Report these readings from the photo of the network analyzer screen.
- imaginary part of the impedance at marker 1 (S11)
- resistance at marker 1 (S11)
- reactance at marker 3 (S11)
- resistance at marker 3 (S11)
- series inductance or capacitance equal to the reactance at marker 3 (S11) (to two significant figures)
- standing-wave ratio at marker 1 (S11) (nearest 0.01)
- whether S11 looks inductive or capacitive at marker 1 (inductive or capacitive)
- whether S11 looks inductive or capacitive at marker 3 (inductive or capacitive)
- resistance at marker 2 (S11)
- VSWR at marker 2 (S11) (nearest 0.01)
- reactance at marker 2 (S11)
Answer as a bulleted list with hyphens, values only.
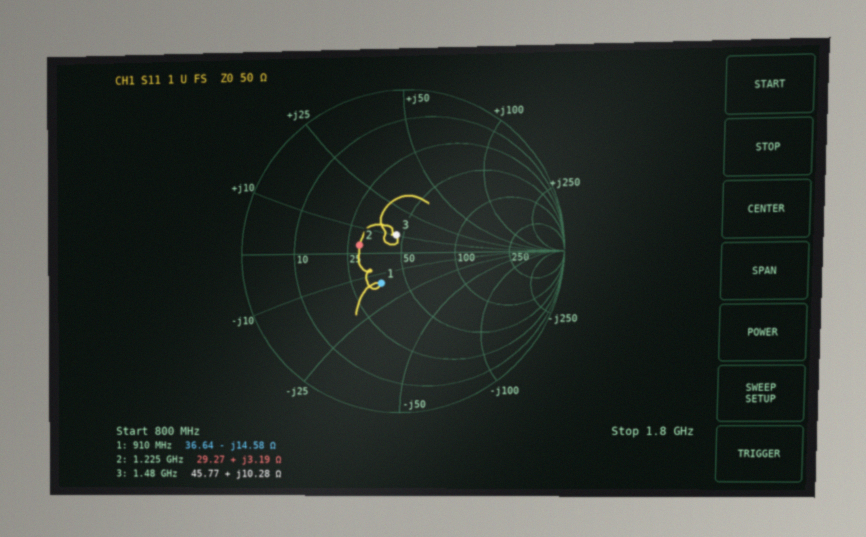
- -14.58 Ω
- 36.64 Ω
- +10.28 Ω
- 45.77 Ω
- 1.1 nH
- 1.58
- capacitive
- inductive
- 29.27 Ω
- 1.72
- +3.19 Ω
